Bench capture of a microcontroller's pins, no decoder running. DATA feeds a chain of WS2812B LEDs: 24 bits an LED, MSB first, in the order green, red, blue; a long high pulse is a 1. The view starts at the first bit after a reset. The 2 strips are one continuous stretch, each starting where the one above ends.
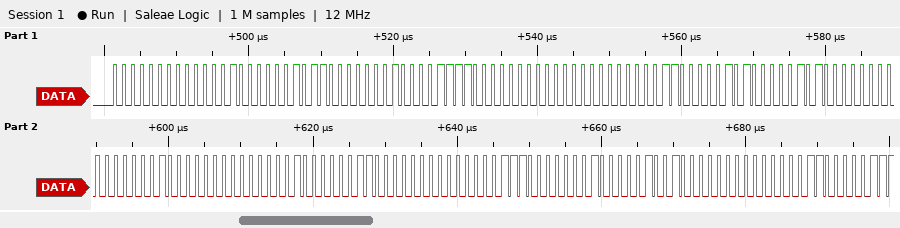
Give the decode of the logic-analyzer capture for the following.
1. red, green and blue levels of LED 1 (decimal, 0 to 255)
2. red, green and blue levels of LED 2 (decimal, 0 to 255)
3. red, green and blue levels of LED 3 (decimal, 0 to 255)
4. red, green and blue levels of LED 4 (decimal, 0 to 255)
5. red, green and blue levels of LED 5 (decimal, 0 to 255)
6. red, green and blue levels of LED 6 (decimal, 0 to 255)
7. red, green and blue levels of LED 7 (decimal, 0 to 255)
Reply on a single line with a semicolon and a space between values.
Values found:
4, 0, 11; 15, 1, 0; 6, 0, 10; 0, 10, 2; 4, 0, 12; 14, 0, 2; 0, 9, 3
